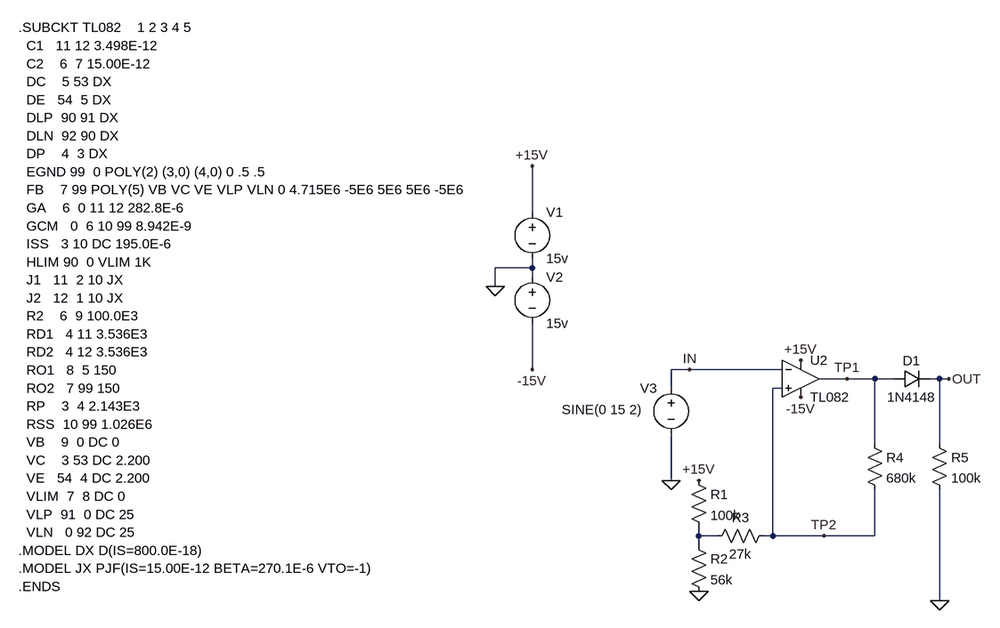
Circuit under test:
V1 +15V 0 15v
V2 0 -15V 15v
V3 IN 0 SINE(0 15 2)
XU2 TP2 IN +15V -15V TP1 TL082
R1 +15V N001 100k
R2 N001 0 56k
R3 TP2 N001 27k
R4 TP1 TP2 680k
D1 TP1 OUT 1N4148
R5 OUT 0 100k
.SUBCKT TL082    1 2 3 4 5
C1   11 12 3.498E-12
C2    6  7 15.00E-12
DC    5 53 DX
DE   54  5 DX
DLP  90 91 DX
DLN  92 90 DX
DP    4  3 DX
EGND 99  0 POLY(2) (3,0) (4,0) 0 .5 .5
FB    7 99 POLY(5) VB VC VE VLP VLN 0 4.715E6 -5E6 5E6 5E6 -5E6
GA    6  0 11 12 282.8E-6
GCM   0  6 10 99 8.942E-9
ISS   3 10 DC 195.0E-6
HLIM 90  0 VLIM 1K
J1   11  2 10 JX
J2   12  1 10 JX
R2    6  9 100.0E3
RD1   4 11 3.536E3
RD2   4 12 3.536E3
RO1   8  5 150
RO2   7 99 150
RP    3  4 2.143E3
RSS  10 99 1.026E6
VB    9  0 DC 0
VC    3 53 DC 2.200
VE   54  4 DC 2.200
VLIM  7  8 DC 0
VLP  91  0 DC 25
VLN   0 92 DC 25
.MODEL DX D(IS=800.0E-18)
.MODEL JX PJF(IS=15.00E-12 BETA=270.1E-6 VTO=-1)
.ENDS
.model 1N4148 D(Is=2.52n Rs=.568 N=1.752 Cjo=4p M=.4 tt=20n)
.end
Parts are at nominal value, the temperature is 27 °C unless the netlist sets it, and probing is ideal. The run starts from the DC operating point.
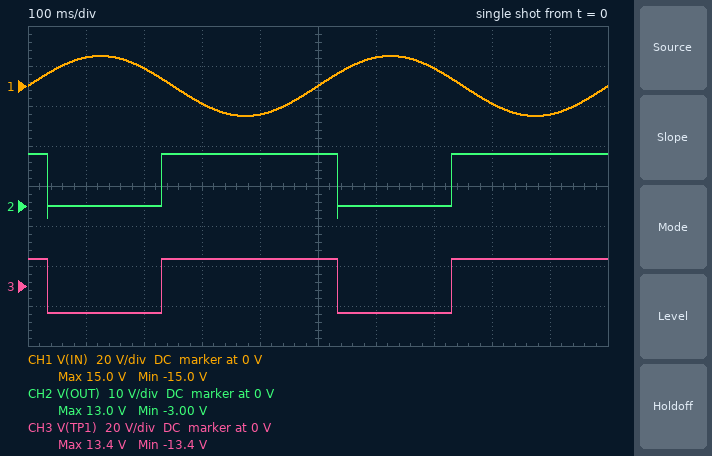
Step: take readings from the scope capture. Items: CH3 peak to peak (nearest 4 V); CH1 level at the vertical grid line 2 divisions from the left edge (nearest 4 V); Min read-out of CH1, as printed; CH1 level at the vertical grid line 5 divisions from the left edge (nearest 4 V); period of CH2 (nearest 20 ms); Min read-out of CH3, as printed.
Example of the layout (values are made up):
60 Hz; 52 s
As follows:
28 V; 8 V; -15.0 V; 0 V; 500 ms; -13.4 V
